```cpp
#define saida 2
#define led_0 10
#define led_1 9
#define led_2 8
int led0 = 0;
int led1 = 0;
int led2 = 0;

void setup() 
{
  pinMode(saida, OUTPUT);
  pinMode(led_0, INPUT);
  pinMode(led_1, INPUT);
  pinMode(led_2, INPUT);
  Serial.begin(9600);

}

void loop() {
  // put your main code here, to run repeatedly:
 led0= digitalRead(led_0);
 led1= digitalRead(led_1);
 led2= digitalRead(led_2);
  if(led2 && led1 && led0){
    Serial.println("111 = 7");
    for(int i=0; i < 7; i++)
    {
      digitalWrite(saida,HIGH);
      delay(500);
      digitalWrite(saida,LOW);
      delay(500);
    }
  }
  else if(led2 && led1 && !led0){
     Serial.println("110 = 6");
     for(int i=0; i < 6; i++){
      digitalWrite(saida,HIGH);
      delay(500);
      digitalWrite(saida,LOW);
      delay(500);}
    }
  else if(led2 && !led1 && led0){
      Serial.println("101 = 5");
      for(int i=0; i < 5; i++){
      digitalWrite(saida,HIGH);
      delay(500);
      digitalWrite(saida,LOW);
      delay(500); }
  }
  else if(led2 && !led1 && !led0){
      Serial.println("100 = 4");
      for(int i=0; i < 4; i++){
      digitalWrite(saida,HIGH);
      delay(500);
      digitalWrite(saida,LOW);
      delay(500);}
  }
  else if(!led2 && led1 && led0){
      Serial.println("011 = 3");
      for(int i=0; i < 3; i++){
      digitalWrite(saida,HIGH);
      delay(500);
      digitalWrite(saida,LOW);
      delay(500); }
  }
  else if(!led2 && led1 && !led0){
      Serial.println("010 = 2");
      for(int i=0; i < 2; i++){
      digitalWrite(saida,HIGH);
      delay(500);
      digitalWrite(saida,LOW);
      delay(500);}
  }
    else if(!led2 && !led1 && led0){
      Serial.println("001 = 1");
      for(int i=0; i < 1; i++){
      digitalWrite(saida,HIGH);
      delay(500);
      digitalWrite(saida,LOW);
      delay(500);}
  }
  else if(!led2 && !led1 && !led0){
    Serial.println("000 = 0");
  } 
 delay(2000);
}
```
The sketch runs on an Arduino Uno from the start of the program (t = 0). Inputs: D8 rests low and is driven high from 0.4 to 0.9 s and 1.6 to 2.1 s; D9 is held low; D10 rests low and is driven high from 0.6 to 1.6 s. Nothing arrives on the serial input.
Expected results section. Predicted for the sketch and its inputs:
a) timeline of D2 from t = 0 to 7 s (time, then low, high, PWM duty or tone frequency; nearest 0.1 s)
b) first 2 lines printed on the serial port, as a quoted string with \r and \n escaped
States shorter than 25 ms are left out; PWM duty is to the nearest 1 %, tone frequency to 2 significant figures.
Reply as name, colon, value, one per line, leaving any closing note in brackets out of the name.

timeline of D2 from t = 0 to 7 s: 0 s low; 2 s high; 2.5 s low; 3 s high; 3.5 s low; 4 s high; 4.5 s low; 5 s high; 5.5 s low
first 2 lines printed on the serial port, as a quoted string with \r and \n escaped: "000 = 0\r\n100 = 4\r\n"
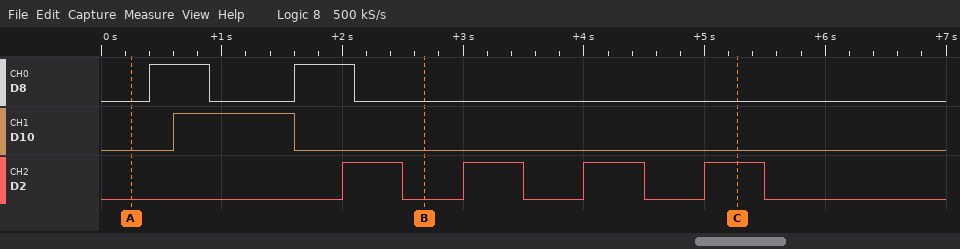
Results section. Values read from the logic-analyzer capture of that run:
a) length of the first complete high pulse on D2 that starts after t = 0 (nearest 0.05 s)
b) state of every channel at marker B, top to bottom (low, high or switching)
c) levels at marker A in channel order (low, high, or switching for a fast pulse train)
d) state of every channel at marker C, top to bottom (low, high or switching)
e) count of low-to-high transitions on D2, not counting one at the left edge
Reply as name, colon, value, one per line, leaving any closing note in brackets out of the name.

length of the first complete high pulse on D2 that starts after t = 0: 0.50 s
state of every channel at marker B, top to bottom: D8 low, D10 low, D2 low
levels at marker A in channel order: D8 low, D10 low, D2 low
state of every channel at marker C, top to bottom: D8 low, D10 low, D2 high
count of low-to-high transitions on D2, not counting one at the left edge: 4
